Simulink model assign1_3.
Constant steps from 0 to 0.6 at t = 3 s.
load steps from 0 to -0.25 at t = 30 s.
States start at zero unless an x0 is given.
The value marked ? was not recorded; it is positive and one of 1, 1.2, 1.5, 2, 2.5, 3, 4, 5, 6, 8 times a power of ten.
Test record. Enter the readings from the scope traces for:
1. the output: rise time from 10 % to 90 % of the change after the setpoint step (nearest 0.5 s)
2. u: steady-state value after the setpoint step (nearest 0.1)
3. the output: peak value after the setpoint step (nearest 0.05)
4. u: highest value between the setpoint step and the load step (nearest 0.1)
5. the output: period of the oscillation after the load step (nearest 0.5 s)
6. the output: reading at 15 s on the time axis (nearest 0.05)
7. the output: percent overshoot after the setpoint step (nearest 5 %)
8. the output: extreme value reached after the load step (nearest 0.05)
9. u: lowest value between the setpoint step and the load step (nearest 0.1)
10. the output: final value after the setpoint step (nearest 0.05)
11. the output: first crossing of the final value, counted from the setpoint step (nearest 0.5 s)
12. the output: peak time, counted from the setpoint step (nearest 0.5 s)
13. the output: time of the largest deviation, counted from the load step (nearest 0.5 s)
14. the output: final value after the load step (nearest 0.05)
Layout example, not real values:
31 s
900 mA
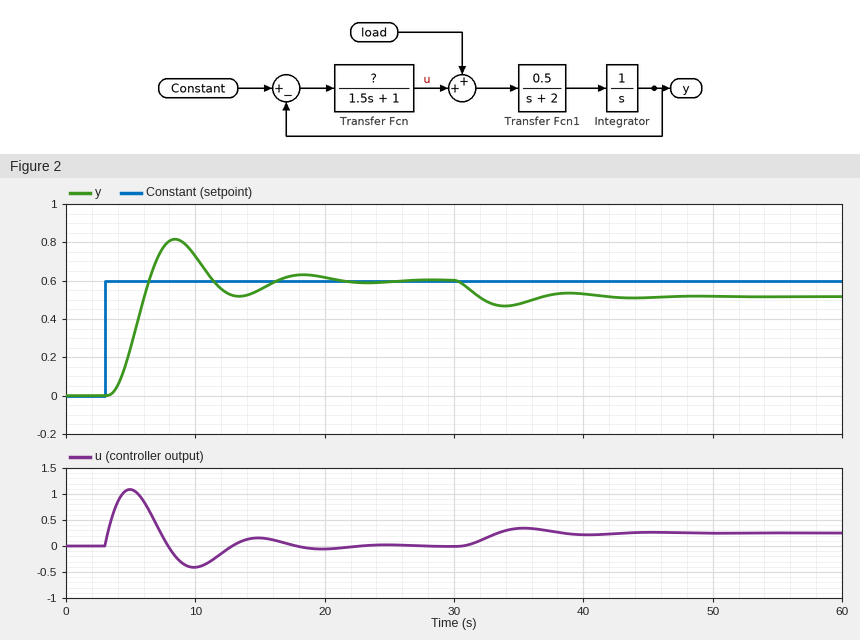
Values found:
2.0 s
0.0
0.80
1.1
10.0 s
0.55
35 %
0.45
-0.4
0.60
3.5 s
5.5 s
4.0 s
0.50
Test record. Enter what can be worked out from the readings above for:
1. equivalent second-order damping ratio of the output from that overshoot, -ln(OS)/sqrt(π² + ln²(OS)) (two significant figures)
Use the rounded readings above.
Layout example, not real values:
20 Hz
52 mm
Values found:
0.32
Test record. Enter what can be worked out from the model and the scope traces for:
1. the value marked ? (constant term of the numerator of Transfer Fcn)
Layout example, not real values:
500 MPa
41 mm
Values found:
3
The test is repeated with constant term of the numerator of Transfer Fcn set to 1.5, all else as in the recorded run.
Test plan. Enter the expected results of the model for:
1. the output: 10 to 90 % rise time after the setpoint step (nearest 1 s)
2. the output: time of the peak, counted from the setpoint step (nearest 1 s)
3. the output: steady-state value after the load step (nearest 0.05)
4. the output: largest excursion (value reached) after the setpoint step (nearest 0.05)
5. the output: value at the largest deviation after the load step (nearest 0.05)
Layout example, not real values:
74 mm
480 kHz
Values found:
4 s
8 s
0.45
0.70
0.40
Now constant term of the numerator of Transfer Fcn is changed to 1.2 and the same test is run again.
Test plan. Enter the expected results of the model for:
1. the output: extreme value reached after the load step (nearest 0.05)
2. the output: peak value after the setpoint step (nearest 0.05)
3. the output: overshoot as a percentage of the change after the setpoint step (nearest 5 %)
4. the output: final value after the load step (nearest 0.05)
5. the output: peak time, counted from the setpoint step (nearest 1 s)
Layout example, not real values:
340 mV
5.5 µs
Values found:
0.35
0.65
10 %
0.40
10 s
